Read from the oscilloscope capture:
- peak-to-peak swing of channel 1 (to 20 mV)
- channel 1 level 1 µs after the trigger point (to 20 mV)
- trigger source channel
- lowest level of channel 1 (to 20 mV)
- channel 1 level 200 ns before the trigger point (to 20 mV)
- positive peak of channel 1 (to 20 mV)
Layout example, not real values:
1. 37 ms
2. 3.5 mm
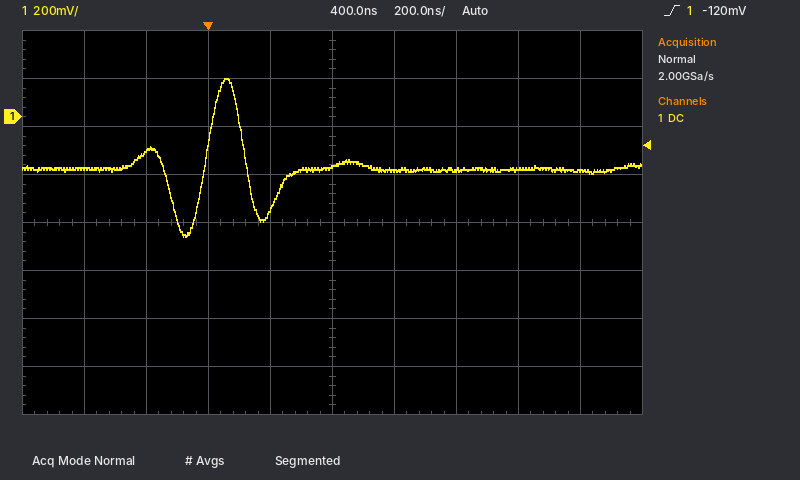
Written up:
1. 660 mV
2. -220 mV
3. channel 1
4. -500 mV
5. -140 mV
6. 160 mV
